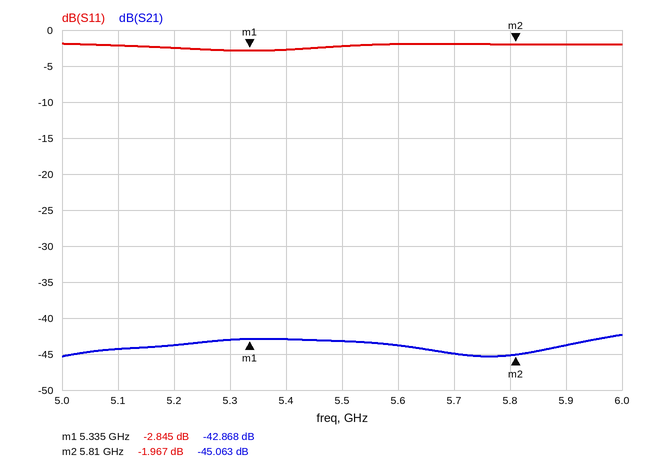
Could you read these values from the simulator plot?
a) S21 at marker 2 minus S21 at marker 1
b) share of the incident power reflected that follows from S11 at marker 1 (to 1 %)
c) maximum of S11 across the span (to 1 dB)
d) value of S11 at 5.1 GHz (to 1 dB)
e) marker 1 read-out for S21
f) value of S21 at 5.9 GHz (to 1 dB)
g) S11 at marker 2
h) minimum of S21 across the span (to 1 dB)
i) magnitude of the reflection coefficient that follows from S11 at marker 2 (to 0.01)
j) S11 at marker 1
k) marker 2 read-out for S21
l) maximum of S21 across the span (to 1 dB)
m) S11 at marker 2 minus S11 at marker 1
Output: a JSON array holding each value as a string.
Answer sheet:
["-2.195 dB", "52 %", "-2 dB", "-2 dB", "-42.868 dB", "-44 dB", "-1.967 dB", "-45 dB", "0.80", "-2.845 dB", "-45.063 dB", "-42 dB", "0.878 dB"]
